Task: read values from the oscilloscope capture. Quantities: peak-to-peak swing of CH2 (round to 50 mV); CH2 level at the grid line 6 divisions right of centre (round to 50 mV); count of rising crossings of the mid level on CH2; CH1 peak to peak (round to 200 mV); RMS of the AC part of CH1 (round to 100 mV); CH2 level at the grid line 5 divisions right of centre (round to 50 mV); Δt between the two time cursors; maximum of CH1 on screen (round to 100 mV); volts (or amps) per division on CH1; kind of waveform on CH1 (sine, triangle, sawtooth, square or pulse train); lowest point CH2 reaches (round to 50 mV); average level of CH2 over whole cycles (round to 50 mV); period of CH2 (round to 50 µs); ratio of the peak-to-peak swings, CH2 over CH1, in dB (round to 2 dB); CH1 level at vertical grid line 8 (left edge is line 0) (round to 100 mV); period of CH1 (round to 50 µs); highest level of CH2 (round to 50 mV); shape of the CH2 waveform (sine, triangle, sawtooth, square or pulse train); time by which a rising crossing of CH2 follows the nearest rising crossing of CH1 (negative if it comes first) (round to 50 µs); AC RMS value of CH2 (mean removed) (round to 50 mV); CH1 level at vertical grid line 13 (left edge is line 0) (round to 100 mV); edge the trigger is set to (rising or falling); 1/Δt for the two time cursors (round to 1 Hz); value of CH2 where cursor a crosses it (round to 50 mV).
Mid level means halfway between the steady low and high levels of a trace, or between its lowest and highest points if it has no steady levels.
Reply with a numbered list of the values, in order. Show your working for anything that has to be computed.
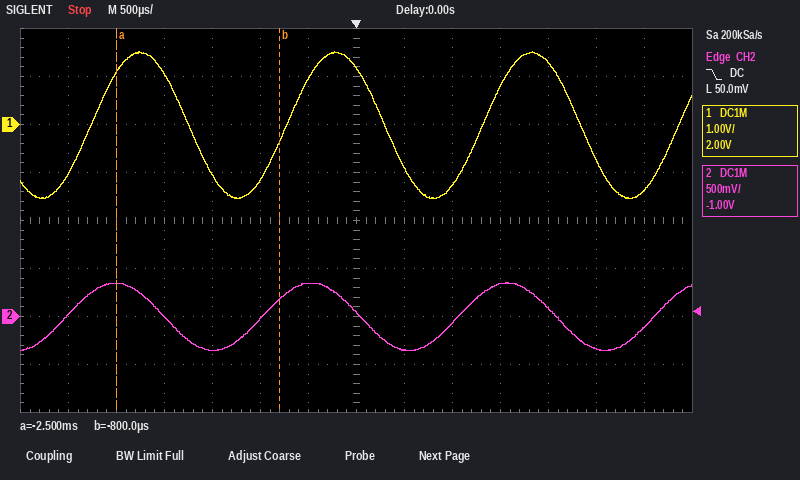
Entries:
1. 350 mV − (-350 mV) = 700 mV
2. -100 mV
3. 4
4. 3.0 V
5. 3.0 V / (2√2) ≈ 1.1 V
6. -350 mV
7. -800 µs − (-2.5 ms) = 1.70 ms
8. 1.5 V
9. 1 V
10. sine
11. -350 mV
12. (350 mV + (-350 mV)) / 2 ≈ 0 mV
13. 2.05 ms
14. 20 log10(700 mV / 3.0 V) ≈ -12.6 dB, so -12 dB to the nearest 2 dB
15. -900 mV
16. 2.05 ms
17. 350 mV
18. sine
19. -250 µs
20. 700 mV / (2√2) ≈ 247 mV, so 250 mV to the nearest 50 mV
21. -1.4 V
22. falling
23. 1 / 1.70 ms ≈ 588 Hz
24. 350 mV
